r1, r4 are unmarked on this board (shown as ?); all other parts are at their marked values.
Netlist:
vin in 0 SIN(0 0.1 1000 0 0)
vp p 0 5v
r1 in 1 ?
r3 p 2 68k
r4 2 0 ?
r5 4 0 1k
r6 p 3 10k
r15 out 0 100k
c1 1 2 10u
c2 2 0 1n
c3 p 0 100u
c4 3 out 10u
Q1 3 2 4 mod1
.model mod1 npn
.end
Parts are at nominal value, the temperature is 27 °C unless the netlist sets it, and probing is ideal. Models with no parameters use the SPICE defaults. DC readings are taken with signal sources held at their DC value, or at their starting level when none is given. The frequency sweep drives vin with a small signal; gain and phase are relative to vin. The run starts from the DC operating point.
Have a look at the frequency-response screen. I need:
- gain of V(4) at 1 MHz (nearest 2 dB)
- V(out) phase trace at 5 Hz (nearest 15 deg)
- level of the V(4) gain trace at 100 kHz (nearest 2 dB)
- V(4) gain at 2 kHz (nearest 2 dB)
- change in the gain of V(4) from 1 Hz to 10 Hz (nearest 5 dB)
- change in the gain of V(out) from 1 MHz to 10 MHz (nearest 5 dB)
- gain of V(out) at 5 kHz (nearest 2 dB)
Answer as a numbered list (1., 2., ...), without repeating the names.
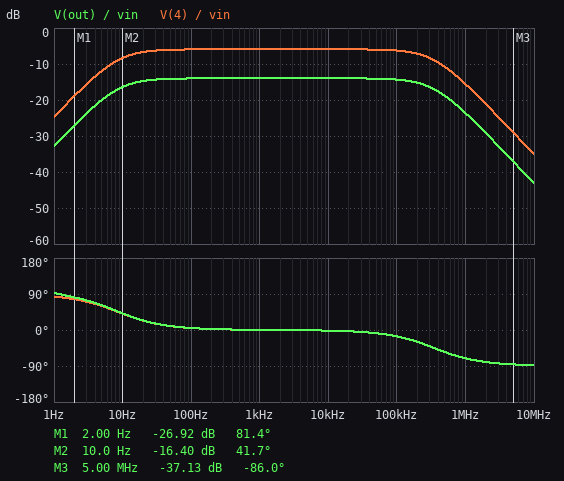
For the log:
1. -16 dB
2. 60 deg
3. -6 dB
4. -6 dB
5. 15 dB
6. -20 dB
7. -14 dB
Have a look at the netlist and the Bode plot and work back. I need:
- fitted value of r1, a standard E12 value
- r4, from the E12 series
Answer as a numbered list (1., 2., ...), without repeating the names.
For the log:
1. 820 Ω
2. 100 kΩ
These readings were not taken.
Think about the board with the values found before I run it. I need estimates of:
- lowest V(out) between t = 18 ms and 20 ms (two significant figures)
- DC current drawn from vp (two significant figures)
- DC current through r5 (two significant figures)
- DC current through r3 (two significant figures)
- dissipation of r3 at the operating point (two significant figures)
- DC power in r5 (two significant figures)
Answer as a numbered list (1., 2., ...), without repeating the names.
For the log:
1. -4.2 mV
2. 500 µA
3. 490 µA
4. 55 µA
5. 210 µW
6. 240 µW
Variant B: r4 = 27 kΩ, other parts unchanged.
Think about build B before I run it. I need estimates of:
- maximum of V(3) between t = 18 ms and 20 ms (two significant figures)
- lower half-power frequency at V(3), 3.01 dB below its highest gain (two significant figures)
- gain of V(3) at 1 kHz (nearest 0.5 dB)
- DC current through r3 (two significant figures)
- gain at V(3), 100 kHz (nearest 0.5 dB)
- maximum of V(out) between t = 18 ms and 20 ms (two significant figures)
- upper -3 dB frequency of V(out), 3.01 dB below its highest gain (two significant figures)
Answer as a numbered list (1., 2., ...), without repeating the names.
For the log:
1. 1.4 V
2. 7.5 Hz
3. 1.0 dB
4. 56 µA
5. 0.5 dB
6. 840 mV
7. 320 kHz
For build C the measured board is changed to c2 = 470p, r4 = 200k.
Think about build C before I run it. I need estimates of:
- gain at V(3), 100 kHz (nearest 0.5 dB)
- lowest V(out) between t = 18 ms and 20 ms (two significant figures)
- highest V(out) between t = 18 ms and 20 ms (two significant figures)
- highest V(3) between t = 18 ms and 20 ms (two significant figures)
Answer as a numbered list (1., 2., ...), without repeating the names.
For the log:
1. -12.5 dB
2. -6.4 mV
3. 130 mV
4. 690 mV
